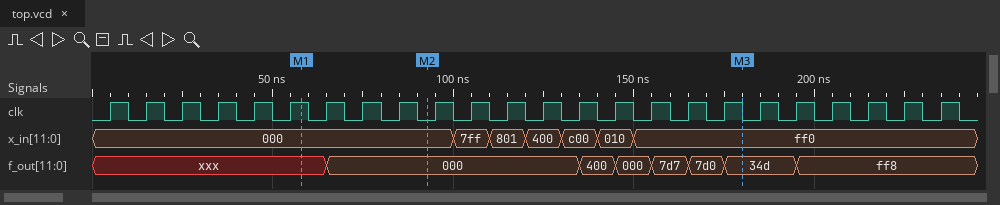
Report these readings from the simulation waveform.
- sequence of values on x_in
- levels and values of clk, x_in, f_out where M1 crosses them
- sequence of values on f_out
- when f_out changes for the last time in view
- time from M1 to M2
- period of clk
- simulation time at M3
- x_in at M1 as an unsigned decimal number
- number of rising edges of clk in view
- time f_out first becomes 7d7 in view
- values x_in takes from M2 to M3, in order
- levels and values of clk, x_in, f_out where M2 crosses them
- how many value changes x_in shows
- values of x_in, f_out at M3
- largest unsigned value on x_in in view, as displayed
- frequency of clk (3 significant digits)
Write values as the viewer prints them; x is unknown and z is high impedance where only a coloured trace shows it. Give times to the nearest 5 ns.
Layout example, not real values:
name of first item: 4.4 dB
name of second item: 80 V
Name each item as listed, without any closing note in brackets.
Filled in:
sequence of values on x_in: 000, 7ff, 801, 400, c00, 010, ff0
levels and values of clk, x_in, f_out where M1 crosses them: clk=1, x_in=000, f_out=xxx
sequence of values on f_out: xxx, 000, 400, 000, 7d7, 7d0, 34d, ff8
when f_out changes for the last time in view: 195 ns
time from M1 to M2: 35 ns
period of clk: 10 ns
simulation time at M3: 180 ns
x_in at M1 as an unsigned decimal number: 0
number of rising edges of clk in view: 24
time f_out first becomes 7d7 in view: 155 ns
values x_in takes from M2 to M3, in order: 000, 7ff, 801, 400, c00, 010, ff0
levels and values of clk, x_in, f_out where M2 crosses them: clk=0, x_in=000, f_out=000
how many value changes x_in shows: 6
values of x_in, f_out at M3: x_in=ff0, f_out=34d
largest unsigned value on x_in in view, as displayed: ff0
frequency of clk: 100 MHz
